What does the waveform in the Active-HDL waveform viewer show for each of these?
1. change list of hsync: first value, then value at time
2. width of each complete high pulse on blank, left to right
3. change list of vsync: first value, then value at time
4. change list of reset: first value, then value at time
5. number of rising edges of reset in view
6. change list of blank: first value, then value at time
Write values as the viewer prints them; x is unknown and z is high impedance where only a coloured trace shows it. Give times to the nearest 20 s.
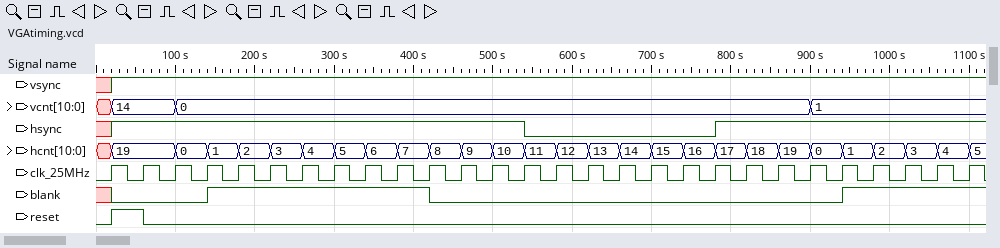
x, 1 at 20 s, 0 at 540 s, 1 at 780 s
280 s
x, 1 at 20 s
0, 1 at 20 s, 0 at 60 s
1
x, 0 at 20 s, 1 at 140 s, 0 at 420 s, 1 at 940 s
